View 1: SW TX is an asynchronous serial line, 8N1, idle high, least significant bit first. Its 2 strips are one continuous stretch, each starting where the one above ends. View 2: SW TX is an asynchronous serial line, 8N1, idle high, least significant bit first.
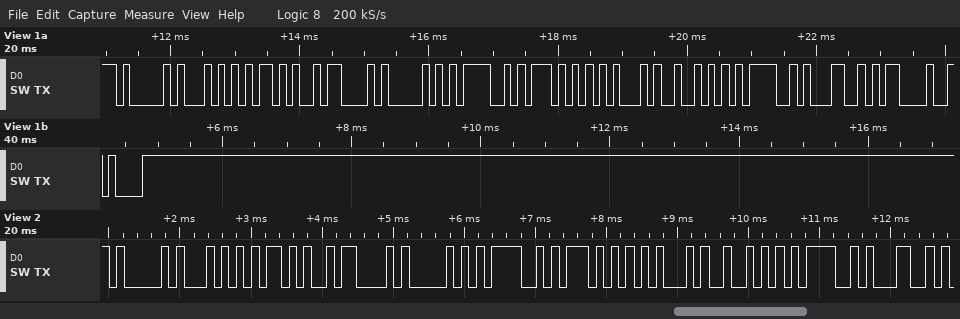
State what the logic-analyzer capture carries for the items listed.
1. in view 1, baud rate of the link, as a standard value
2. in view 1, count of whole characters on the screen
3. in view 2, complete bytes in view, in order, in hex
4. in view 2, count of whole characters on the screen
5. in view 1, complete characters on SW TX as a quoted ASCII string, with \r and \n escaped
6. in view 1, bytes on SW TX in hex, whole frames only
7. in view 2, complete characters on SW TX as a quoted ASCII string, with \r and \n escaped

9600 baud
13
41 54 2B 43 50 4F 57 45 52 3D 31
11
"AT+CPOWER=1\r\n"
41 54 2B 43 50 4F 57 45 52 3D 31 0D 0A
"AT+CPOWER=1"
